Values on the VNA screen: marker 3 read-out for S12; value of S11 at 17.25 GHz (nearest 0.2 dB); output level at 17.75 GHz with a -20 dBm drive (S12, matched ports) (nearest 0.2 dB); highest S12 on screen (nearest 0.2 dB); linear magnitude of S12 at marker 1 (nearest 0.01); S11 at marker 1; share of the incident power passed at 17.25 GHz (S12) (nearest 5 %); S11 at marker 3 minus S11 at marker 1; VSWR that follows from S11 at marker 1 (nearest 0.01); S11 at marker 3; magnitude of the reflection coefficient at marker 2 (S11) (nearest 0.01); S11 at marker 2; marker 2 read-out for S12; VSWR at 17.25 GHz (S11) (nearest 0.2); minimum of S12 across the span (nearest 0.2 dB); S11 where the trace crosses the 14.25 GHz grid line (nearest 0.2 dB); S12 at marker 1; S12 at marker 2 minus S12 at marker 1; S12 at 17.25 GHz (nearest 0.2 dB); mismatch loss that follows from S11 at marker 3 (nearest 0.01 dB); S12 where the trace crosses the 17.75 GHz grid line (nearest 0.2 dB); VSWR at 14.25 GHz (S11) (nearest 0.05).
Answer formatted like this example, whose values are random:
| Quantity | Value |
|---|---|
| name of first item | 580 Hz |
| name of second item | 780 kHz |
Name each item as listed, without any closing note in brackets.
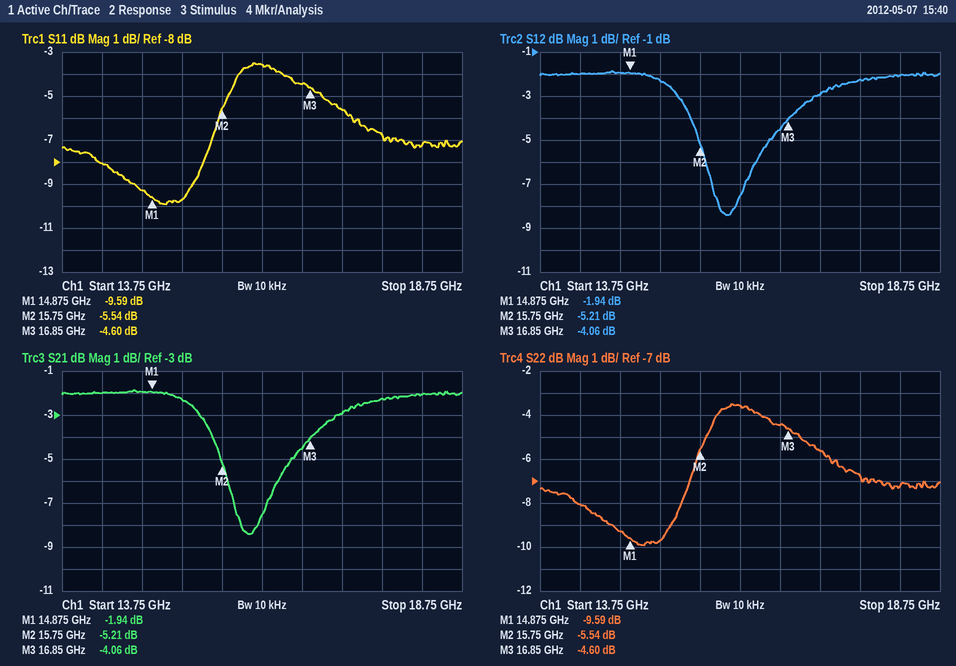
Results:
| Quantity | Value |
|---|---|
| marker 3 read-out for S12 | -4.06 dB |
| value of S11 at 17.25 GHz | -5.6 dB |
| output level at 17.75 GHz with a -20 dBm drive (S12, matched ports) | -22.2 dBm |
| highest S12 on screen | -1.8 dB |
| linear magnitude of S12 at marker 1 | 0.80 |
| S11 at marker 1 | -9.59 dB |
| share of the incident power passed at 17.25 GHz (S12) | 50 % |
| S11 at marker 3 minus S11 at marker 1 | 4.99 dB |
| VSWR that follows from S11 at marker 1 | 1.99 |
| S11 at marker 3 | -4.60 dB |
| magnitude of the reflection coefficient at marker 2 (S11) | 0.53 |
| S11 at marker 2 | -5.54 dB |
| marker 2 read-out for S12 | -5.21 dB |
| VSWR at 17.25 GHz (S11) | 3.2 |
| minimum of S12 across the span | -8.4 dB |
| S11 where the trace crosses the 14.25 GHz grid line | -8.0 dB |
| S12 at marker 1 | -1.94 dB |
| S12 at marker 2 minus S12 at marker 1 | -3.27 dB |
| S12 at 17.25 GHz | -3.0 dB |
| mismatch loss that follows from S11 at marker 3 | 1.85 dB |
| S12 where the trace crosses the 17.75 GHz grid line | -2.2 dB |
| VSWR at 14.25 GHz (S11) | 2.30 |
